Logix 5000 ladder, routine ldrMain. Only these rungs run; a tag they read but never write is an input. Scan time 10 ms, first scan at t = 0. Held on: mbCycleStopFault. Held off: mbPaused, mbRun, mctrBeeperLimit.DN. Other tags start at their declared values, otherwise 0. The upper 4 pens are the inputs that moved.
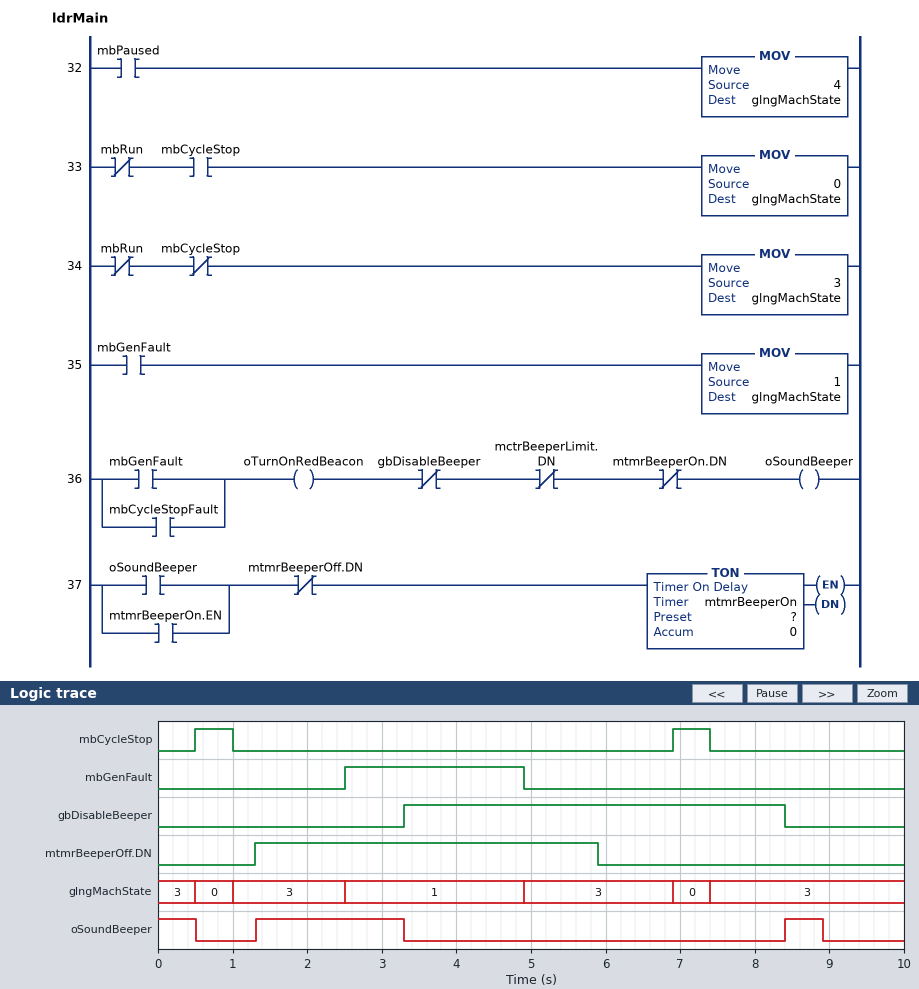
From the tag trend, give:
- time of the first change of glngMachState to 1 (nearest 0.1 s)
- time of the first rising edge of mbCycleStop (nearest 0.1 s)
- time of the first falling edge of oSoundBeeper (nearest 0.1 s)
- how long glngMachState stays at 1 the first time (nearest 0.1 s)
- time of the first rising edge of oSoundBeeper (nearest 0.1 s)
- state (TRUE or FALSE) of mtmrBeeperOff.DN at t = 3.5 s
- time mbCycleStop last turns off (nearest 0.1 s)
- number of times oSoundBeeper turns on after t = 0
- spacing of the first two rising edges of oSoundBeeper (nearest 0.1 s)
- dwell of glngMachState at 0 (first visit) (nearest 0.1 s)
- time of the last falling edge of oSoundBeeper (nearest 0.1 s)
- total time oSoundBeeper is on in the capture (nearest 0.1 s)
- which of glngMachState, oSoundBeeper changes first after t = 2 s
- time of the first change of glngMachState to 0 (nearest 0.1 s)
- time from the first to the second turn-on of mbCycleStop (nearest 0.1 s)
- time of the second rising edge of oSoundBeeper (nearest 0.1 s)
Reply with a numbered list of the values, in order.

1. 2.5 s
2. 0.5 s
3. 0.5 s
4. 2.4 s
5. 1.3 s
6. TRUE
7. 7.4 s
8. 2
9. 7.1 s
10. 0.5 s
11. 8.9 s
12. 3.0 s
13. glngMachState
14. 0.5 s
15. 6.4 s
16. 8.4 s
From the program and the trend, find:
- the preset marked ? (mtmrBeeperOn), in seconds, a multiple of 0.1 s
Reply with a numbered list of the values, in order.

1. 0.5 s
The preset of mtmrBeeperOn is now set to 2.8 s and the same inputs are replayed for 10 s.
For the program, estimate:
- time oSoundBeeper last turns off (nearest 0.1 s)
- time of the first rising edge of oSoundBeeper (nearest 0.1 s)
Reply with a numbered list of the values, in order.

1. 3.3 s
2. 8.4 s
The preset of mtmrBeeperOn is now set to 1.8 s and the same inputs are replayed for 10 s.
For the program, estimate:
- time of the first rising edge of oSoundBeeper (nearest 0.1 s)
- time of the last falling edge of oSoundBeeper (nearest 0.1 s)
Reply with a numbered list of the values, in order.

1. 8.4 s
2. 3.3 s
